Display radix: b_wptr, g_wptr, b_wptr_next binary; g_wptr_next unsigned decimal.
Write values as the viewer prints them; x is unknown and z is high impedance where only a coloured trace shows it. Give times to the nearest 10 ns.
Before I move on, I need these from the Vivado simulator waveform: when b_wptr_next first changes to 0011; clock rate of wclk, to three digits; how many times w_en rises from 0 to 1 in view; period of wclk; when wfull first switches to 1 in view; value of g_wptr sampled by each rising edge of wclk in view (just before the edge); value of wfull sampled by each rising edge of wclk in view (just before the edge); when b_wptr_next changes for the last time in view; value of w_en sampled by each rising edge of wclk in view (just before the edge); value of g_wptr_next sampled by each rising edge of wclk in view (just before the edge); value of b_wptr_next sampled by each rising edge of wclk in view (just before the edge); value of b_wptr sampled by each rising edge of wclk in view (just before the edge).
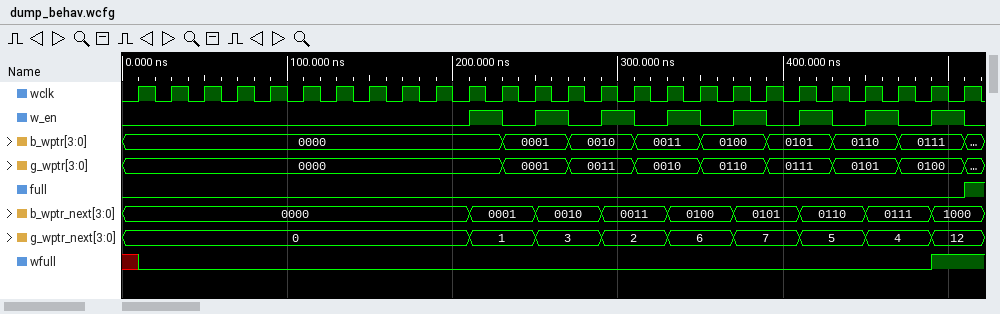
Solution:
290 ns
50.0 MHz
8
20 ns
490 ns
0000, 0000, 0000, 0000, 0000, 0000, 0000, 0000, 0000, 0000, 0000, 0000, 0001, 0001, 0011, 0011, 0010, 0010, 0110, 0110, 0111, 0111, 0101, 0101, 0100, 0100
x 0 0 0 0 0 0 0 0 0 0 0 0 0 0 0 0 0 0 0 0 0 0 0 0 1
490 ns
0 0 0 0 0 0 0 0 0 0 0 1 0 1 0 1 0 1 0 1 0 1 0 1 0 1
0, 0, 0, 0, 0, 0, 0, 0, 0, 0, 0, 1, 1, 3, 3, 2, 2, 6, 6, 7, 7, 5, 5, 4, 4, 12
0000, 0000, 0000, 0000, 0000, 0000, 0000, 0000, 0000, 0000, 0000, 0001, 0001, 0010, 0010, 0011, 0011, 0100, 0100, 0101, 0101, 0110, 0110, 0111, 0111, 1000
0000, 0000, 0000, 0000, 0000, 0000, 0000, 0000, 0000, 0000, 0000, 0000, 0001, 0001, 0010, 0010, 0011, 0011, 0100, 0100, 0101, 0101, 0110, 0110, 0111, 0111
